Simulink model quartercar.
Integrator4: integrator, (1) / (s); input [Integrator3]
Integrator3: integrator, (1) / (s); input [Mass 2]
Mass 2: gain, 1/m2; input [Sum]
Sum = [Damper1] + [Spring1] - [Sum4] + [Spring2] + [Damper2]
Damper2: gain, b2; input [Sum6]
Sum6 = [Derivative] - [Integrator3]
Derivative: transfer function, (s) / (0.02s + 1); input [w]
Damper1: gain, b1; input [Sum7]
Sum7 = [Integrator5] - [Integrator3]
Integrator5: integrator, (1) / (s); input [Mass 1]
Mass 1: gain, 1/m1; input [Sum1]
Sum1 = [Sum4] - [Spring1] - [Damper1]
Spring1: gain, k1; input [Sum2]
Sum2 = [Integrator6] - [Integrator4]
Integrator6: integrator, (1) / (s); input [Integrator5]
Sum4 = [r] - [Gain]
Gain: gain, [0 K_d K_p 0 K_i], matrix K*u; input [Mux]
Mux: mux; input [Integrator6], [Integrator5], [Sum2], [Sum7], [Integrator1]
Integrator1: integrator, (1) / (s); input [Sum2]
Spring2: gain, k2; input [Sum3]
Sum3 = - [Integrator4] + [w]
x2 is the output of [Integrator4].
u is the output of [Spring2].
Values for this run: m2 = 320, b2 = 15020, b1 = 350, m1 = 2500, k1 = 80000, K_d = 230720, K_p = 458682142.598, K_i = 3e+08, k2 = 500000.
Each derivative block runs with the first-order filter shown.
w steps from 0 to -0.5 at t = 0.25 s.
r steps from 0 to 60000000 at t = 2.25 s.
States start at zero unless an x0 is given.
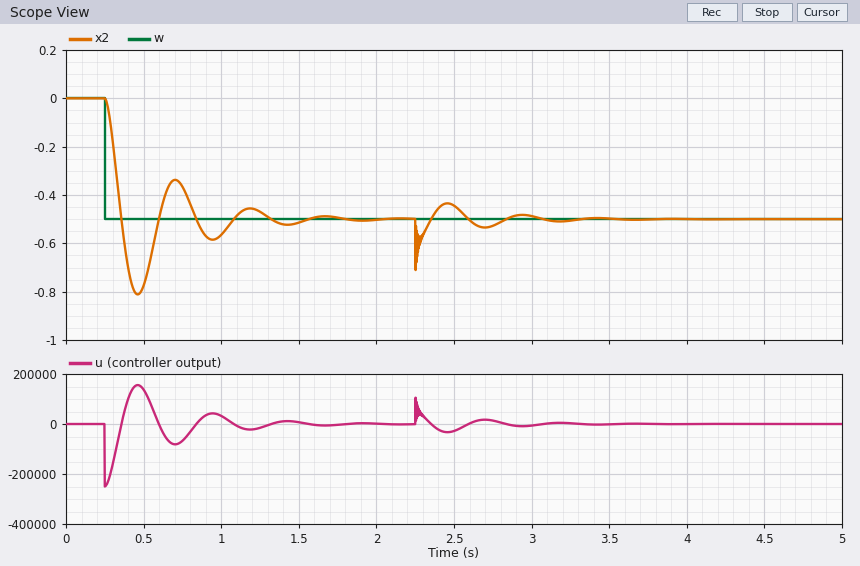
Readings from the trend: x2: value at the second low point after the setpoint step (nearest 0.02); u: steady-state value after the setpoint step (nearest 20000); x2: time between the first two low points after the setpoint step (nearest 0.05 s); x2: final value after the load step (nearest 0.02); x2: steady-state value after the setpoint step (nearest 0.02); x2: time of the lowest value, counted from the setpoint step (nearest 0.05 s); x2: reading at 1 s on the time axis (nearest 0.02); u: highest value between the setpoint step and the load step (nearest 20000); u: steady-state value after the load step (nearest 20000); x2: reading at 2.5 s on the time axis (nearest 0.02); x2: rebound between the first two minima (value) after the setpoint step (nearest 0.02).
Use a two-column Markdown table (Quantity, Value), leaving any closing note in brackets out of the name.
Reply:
| Quantity | Value |
|---|---|
| x2: value at the second low point after the setpoint step | -0.58 |
| u: steady-state value after the setpoint step | 0 |
| x2: time between the first two low points after the setpoint step | 0.50 s |
| x2: final value after the load step | -0.50 |
| x2: steady-state value after the setpoint step | -0.50 |
| x2: time of the lowest value, counted from the setpoint step | 0.20 s |
| x2: reading at 1 s on the time axis | -0.56 |
| u: highest value between the setpoint step and the load step | 160000 |
| u: steady-state value after the load step | 0 |
| x2: reading at 2.5 s on the time axis | -0.44 |
| x2: rebound between the first two minima (value) after the setpoint step | -0.34 |
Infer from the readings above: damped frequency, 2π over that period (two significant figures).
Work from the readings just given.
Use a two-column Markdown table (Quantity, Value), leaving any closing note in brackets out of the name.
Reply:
| Quantity | Value |
|---|---|
| damped frequency, 2π over that period | 13 rad/s |
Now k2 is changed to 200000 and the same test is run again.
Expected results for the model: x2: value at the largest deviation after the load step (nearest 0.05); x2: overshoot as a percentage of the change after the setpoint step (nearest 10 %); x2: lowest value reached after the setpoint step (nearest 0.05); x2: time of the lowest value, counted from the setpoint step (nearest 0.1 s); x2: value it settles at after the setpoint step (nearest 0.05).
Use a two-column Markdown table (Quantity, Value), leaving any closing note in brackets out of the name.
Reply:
| Quantity | Value |
|---|---|
| x2: value at the largest deviation after the load step | -0.70 |
| x2: overshoot as a percentage of the change after the setpoint step | 50 % |
| x2: lowest value reached after the setpoint step | -0.75 |
| x2: time of the lowest value, counted from the setpoint step | 0.3 s |
| x2: value it settles at after the setpoint step | -0.50 |
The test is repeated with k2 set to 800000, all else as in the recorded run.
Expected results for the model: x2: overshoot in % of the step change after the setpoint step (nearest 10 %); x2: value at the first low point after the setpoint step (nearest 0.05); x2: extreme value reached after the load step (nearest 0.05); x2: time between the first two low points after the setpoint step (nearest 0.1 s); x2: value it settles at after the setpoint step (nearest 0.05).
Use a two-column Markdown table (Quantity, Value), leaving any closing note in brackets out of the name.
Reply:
| Quantity | Value |
|---|---|
| x2: overshoot in % of the step change after the setpoint step | 70 % |
| x2: value at the first low point after the setpoint step | -0.85 |
| x2: extreme value reached after the load step | -0.70 |
| x2: time between the first two low points after the setpoint step | 0.4 s |
| x2: value it settles at after the setpoint step | -0.50 |
